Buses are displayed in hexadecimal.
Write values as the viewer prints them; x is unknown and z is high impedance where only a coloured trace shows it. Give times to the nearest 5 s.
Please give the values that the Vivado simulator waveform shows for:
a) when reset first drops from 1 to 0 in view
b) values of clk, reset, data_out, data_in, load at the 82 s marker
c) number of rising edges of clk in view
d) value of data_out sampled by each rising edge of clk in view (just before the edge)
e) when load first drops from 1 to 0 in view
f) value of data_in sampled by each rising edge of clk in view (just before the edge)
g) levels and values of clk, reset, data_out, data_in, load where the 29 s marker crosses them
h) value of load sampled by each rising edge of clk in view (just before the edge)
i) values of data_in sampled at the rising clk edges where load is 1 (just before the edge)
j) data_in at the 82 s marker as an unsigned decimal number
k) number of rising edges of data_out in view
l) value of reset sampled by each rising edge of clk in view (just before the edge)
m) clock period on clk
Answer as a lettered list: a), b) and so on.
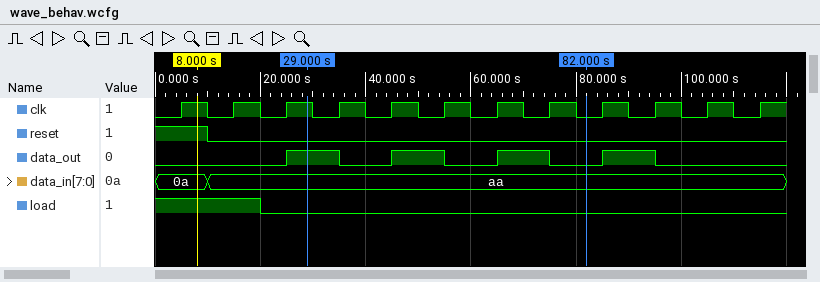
a) 10 s
b) clk=0, reset=0, data_out=0, data_in=aa, load=0
c) 12
d) 0 0 0 1 0 1 0 1 0 1 0 0
e) 20 s
f) 0a, aa, aa, aa, aa, aa, aa, aa, aa, aa, aa, aa
g) clk=1, reset=0, data_out=1, data_in=aa, load=0
h) 1 1 0 0 0 0 0 0 0 0 0 0
i) 0a, aa
j) 170
k) 4
l) 1 0 0 0 0 0 0 0 0 0 0 0
m) 10 s
